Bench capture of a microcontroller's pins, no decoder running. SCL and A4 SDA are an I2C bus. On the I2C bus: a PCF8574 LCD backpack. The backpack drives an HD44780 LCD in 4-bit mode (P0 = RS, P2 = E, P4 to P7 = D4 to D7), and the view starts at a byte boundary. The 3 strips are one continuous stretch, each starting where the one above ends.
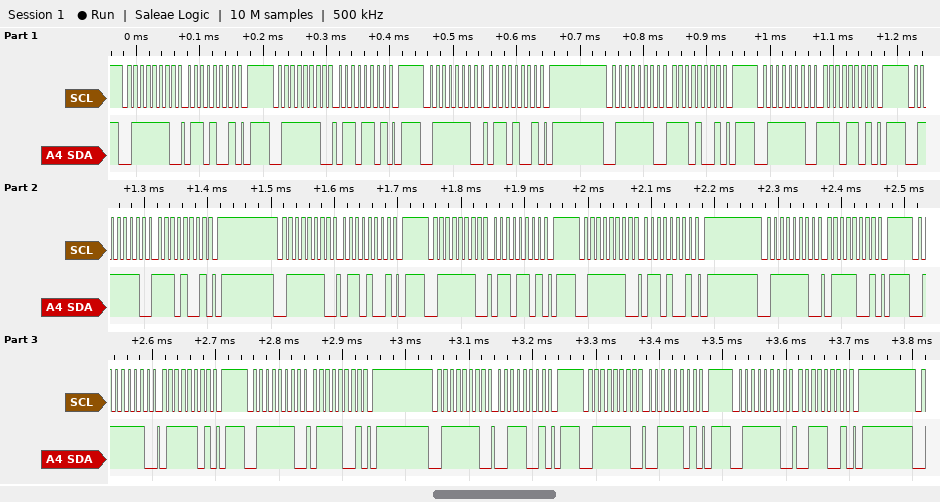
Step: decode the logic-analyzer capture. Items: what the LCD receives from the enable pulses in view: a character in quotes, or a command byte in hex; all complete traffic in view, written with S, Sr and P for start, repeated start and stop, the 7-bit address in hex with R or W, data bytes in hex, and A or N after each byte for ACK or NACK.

'n' 'g'
S 3FW A 69 A P S 3FW A 6D A P S 3FW A 69 A P S 3FW A E9 A P S 3FW A ED A P S 3FW A E9 A P S 3FW A 69 A P S 3FW A 6D A P S 3FW A 69 A P S 3FW A 79 A P S 3FW A 7D A P S 3FW A 79 A P S 3FW A 39 A P S 3FW A 3D A P S 3FW A 39 A P
